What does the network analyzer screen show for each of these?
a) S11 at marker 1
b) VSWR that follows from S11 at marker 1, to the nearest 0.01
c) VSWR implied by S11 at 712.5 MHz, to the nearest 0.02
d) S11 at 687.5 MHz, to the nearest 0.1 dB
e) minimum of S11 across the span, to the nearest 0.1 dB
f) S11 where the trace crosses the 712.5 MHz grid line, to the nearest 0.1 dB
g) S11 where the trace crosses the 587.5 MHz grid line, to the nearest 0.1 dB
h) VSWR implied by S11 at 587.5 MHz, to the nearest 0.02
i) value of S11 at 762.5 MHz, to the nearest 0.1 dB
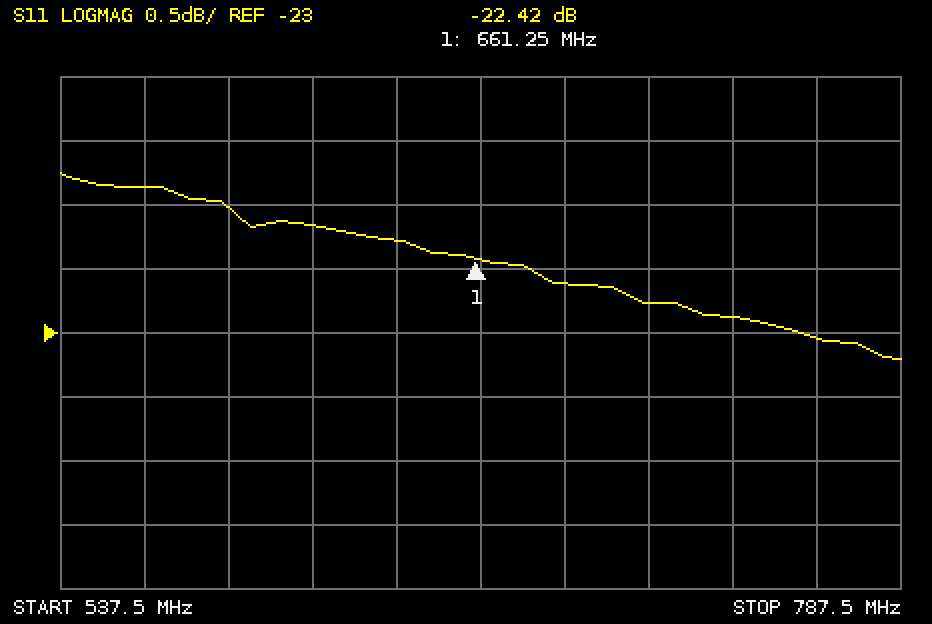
-22.42 dB
1.16
1.16
-22.6 dB
-23.2 dB
-22.8 dB
-22.0 dB
1.18
-23.0 dB
